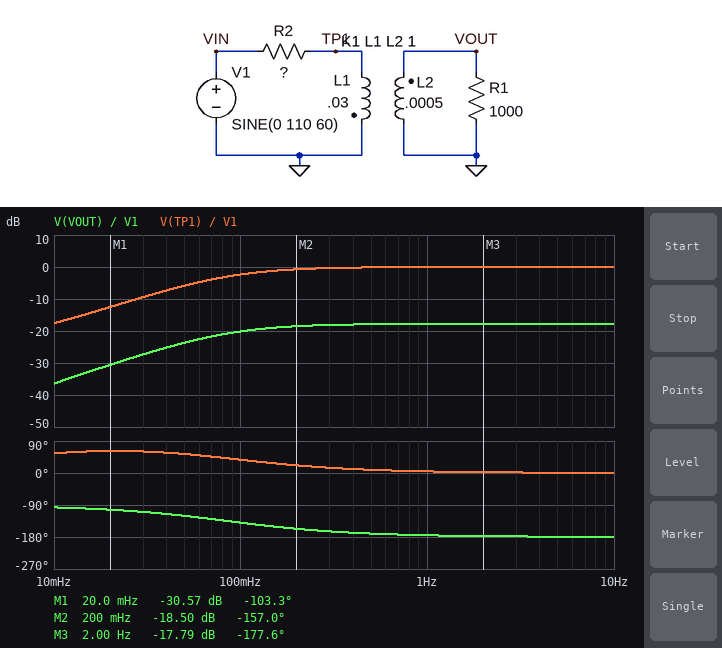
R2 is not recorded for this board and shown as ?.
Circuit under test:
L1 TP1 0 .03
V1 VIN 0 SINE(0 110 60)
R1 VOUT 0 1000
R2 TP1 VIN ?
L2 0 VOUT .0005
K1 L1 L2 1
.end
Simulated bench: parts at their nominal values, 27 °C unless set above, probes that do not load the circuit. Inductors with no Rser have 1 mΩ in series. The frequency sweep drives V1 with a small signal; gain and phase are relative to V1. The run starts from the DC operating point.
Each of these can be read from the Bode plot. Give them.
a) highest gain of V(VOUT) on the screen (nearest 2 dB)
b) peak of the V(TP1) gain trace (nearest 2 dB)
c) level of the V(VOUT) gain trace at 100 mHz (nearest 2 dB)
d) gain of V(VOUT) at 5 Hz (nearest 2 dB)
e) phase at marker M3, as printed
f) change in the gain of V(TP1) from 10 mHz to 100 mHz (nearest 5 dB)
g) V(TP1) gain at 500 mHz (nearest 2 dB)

-18 dB
0 dB
-20 dB
-18 dB
-177.6 deg
15 dB
0 dB
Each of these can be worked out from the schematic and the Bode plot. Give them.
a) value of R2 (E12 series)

0.015 Ω
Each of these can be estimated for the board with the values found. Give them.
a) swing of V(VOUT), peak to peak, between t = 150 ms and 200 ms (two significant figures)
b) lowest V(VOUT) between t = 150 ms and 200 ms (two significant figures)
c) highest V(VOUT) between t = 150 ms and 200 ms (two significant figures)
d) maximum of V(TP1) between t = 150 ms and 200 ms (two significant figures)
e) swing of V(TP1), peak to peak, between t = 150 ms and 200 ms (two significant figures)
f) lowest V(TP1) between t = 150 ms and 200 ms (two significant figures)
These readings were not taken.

28 V
-14 V
14 V
110 V
220 V
-110 V
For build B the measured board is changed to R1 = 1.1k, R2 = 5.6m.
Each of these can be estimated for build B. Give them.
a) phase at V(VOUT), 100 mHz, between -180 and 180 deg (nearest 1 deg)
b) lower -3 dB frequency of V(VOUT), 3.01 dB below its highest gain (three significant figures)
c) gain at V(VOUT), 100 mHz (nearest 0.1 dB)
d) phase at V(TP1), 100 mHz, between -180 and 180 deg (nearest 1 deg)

-161 deg
35.0 mHz
-18.3 dB
16 deg
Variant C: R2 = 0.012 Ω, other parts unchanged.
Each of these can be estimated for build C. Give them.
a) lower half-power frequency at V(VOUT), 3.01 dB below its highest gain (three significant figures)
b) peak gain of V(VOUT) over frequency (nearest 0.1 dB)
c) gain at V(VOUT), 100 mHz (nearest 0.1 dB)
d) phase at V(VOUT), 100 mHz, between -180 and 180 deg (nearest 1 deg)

69.0 mHz
-17.8 dB
-19.5 dB
-145 deg
